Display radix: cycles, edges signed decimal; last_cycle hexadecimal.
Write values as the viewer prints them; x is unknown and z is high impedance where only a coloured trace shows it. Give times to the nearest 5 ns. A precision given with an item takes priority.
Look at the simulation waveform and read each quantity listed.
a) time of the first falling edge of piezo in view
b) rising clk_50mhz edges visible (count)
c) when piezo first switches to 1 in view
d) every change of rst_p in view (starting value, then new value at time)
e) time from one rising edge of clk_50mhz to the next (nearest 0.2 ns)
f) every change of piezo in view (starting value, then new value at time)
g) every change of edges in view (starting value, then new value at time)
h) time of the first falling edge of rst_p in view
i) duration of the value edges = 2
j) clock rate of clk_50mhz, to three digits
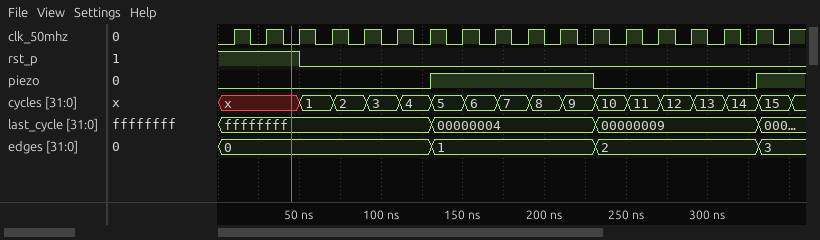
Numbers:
230 ns
18
130 ns
1, 0 at 50 ns
20 ns
0, 1 at 130 ns, 0 at 230 ns, 1 at 330 ns
0, 1 at 130 ns, 2 at 230 ns, 3 at 330 ns
50 ns
100 ns
50.0 MHz
